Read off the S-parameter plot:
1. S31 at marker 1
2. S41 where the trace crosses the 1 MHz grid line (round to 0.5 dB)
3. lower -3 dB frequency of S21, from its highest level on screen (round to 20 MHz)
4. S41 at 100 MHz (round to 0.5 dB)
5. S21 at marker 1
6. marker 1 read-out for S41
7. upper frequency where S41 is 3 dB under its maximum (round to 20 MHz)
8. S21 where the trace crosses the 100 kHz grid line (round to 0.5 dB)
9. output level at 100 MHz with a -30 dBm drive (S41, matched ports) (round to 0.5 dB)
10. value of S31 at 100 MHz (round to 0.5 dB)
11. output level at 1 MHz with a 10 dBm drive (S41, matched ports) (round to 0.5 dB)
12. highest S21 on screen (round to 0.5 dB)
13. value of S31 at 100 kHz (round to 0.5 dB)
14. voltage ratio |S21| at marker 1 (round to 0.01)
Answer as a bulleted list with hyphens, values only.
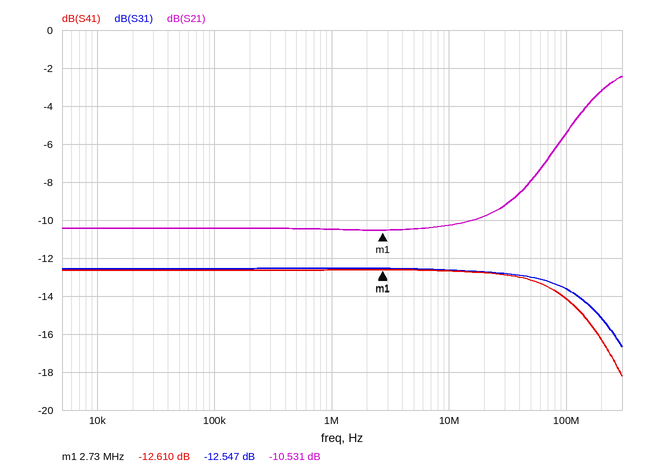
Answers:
- -12.547 dB
- -12.5 dB
- 100 MHz
- -14.0 dB
- -10.531 dB
- -12.610 dB
- 160 MHz
- -10.5 dB
- -44.0 dBm
- -13.5 dB
- -2.5 dBm
- -2.5 dB
- -12.5 dB
- 0.30
